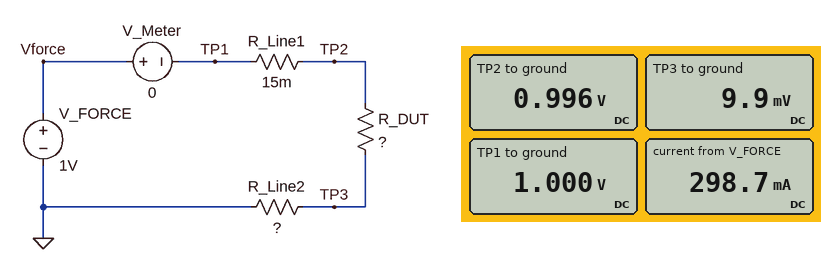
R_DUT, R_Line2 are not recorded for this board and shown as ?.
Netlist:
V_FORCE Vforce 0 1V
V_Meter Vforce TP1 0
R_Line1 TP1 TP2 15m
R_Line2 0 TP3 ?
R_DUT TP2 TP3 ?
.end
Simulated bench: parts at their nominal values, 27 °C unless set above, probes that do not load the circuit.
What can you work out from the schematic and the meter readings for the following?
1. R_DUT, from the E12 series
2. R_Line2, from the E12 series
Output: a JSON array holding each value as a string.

["3.3 Ω", "0.033 Ω"]
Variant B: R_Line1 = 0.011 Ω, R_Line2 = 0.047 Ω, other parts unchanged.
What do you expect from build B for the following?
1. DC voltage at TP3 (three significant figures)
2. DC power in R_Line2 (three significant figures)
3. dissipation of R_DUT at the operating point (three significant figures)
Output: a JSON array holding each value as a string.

["14.0 mV", "4.17 mW", "293 mW"]
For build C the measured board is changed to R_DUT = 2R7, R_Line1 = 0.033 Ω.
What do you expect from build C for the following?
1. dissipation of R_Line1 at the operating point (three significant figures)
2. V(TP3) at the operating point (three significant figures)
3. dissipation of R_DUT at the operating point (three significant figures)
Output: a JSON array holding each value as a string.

["4.31 mW", "11.9 mV", "353 mW"]
